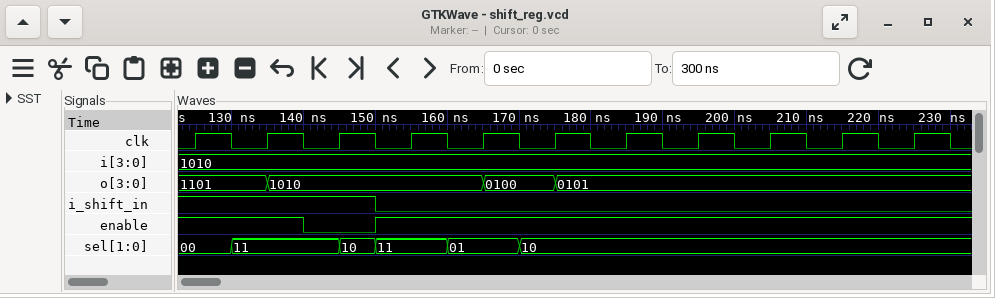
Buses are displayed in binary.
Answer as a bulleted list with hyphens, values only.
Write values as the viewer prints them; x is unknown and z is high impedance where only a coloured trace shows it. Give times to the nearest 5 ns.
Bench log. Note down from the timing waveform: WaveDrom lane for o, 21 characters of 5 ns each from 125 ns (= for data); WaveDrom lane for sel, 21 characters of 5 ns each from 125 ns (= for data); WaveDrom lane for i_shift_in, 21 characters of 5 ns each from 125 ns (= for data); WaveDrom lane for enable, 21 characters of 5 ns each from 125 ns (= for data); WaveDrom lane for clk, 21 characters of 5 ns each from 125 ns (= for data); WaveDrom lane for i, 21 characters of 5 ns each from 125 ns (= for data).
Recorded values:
- {name: 'o', wave: '=.=.....=.=..........', data: '1101 1010 0100 0101'}
- {name: 'sel', wave: '==..==.=.=...........', data: '00 11 10 11 01 10'}
- {name: 'i_shift_in', wave: '1....0...............'}
- {name: 'enable', wave: '1..0.1...............'}
- {name: 'clk', wave: '101010101010101010101'}
- {name: 'i', wave: '=....................', data: '1010'}
